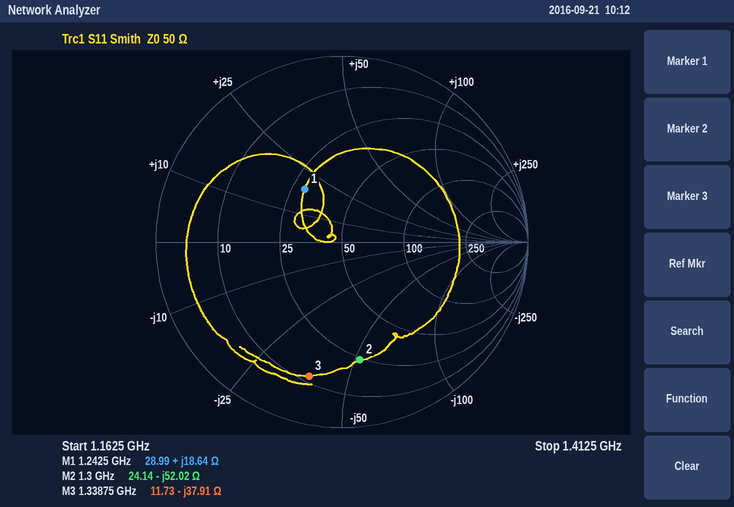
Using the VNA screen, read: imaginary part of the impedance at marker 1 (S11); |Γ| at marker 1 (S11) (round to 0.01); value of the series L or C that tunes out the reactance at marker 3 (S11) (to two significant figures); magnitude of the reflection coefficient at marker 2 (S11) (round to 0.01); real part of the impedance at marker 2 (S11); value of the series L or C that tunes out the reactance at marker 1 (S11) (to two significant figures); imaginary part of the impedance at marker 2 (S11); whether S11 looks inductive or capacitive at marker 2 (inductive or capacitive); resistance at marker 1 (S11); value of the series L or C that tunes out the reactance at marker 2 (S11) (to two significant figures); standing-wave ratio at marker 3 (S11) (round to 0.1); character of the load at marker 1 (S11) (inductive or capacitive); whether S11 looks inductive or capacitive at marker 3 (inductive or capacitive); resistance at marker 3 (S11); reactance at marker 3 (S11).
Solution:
+18.64 Ω
0.35
4.5 nH
0.64
24.14 Ω
6.9 pF
-52.02 Ω
capacitive
28.99 Ω
6.4 nH
6.8
inductive
capacitive
11.73 Ω
-37.91 Ω
